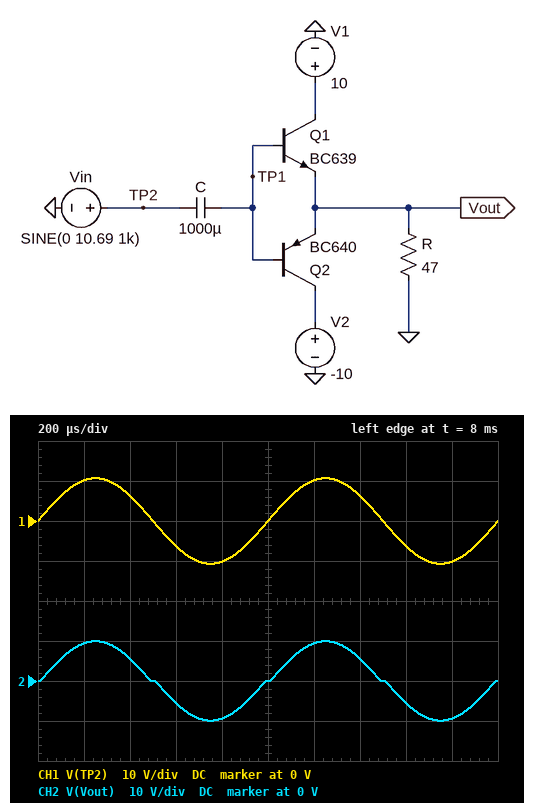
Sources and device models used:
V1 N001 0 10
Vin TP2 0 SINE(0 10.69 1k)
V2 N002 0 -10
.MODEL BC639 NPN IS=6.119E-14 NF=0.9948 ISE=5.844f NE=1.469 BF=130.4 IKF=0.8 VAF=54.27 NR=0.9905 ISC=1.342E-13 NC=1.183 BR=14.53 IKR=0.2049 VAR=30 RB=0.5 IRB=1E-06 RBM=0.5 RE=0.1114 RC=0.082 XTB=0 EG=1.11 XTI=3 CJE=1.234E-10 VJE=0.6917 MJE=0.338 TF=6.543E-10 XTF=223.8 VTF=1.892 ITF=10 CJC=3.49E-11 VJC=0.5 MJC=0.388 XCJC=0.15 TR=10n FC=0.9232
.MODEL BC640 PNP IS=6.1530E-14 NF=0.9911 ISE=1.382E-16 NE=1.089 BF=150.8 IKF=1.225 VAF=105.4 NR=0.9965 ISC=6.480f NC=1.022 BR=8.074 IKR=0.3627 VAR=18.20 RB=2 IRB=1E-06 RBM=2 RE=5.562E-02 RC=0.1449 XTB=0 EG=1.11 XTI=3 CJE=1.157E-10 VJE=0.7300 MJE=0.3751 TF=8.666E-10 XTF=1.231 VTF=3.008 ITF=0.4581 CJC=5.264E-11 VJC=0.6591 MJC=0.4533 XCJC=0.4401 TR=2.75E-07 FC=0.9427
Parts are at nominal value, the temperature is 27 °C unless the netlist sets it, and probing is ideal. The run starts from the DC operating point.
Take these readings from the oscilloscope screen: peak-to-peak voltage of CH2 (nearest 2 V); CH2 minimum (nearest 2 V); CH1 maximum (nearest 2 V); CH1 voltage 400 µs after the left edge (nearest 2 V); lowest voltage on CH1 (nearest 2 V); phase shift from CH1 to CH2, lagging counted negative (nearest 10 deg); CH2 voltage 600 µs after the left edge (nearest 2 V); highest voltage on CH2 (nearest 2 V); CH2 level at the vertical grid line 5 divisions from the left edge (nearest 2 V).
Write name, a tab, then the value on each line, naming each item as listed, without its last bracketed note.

peak-to-peak voltage of CH2	20 V
CH2 minimum	-10 V
CH1 maximum	10 V
CH1 voltage 400 µs after the left edge	6 V
lowest voltage on CH1	-10 V
phase shift from CH1 to CH2, lagging counted negative	0 deg
CH2 voltage 600 µs after the left edge	-6 V
highest voltage on CH2	10 V
CH2 level at the vertical grid line 5 divisions from the left edge	0 V
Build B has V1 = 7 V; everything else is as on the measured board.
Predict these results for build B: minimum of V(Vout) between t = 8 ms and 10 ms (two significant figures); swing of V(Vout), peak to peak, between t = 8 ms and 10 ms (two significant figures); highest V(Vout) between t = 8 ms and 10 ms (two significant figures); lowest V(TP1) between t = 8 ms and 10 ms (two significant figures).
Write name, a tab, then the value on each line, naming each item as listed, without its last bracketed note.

minimum of V(Vout) between t = 8 ms and 10 ms	-10 V
swing of V(Vout), peak to peak, between t = 8 ms and 10 ms	17 V
highest V(Vout) between t = 8 ms and 10 ms	7.1 V
lowest V(TP1) between t = 8 ms and 10 ms	-13 V
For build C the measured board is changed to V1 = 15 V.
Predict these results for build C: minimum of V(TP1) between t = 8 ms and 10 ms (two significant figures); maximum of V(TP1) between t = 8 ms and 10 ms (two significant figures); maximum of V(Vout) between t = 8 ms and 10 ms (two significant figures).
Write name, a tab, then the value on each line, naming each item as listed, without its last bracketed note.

minimum of V(TP1) between t = 8 ms and 10 ms	-10 V
maximum of V(TP1) between t = 8 ms and 10 ms	11 V
maximum of V(Vout) between t = 8 ms and 10 ms	10 V
